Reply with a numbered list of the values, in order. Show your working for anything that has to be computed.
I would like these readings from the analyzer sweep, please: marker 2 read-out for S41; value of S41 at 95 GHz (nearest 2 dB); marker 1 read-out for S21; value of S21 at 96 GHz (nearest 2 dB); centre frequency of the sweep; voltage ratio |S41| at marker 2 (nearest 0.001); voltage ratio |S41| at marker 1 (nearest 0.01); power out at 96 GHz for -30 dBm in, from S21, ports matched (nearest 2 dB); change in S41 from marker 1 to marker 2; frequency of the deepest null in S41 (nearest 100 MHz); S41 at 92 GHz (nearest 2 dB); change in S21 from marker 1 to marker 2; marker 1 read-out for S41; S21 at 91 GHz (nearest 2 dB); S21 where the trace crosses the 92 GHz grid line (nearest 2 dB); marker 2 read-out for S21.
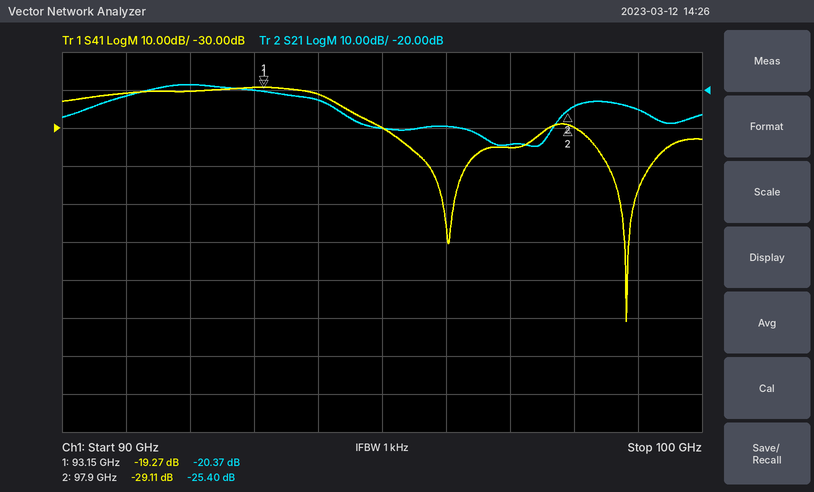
1. -29.11 dB
2. -30 dB
3. -20.37 dB
4. -30 dB
5. 95 GHz
6. 10^(-29.11/20) ≈ 0.035
7. 10^(-19.27/20) ≈ 0.11
8. -30 dBm + (-30 dB) = -60 dBm
9. -29.11 − (-19.27) = -9.84 dB
10. 98.8 GHz
11. -20 dB
12. -25.4 − (-20.37) = -5.03 dB
13. -19.27 dB
14. -22 dB
15. -18 dB
16. -25.40 dB
